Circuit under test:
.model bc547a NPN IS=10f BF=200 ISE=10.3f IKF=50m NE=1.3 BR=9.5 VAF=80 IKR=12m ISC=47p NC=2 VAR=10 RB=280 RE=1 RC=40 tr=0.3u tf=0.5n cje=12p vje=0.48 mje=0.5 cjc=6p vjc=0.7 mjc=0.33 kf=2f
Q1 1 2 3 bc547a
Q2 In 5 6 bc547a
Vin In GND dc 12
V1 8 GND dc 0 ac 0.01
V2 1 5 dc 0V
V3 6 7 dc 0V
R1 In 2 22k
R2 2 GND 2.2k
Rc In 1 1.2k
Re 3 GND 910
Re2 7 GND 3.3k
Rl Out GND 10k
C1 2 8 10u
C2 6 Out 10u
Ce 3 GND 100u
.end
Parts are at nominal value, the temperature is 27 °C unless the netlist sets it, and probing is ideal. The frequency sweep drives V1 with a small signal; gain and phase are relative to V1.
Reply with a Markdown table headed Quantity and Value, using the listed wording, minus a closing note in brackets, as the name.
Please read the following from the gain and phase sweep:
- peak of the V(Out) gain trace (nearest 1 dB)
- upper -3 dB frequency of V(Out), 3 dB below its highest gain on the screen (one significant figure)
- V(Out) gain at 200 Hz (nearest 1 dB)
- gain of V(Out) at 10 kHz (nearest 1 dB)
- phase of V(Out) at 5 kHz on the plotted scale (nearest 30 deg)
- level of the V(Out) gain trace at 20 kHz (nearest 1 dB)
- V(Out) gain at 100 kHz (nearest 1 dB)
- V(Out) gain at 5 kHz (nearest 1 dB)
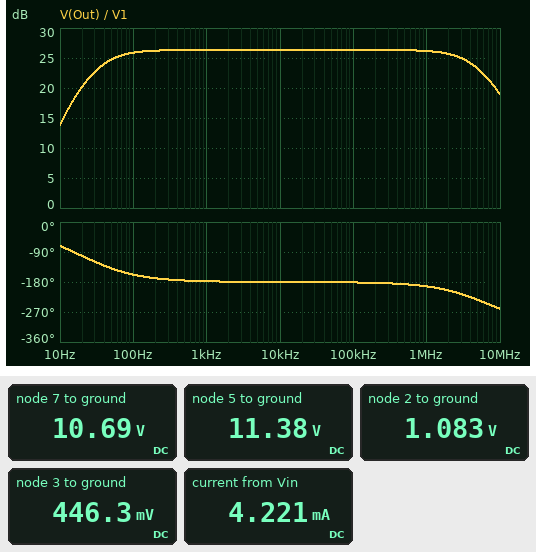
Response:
| Quantity | Value |
|---|---|
| peak of the V(Out) gain trace | 26 dB |
| upper -3 dB frequency of V(Out), 3 dB below its highest gain on the screen | 5 MHz |
| V(Out) gain at 200 Hz | 26 dB |
| gain of V(Out) at 10 kHz | 26 dB |
| phase of V(Out) at 5 kHz on the plotted scale | -180 deg |
| level of the V(Out) gain trace at 20 kHz | 26 dB |
| V(Out) gain at 100 kHz | 26 dB |
| V(Out) gain at 5 kHz | 26 dB |
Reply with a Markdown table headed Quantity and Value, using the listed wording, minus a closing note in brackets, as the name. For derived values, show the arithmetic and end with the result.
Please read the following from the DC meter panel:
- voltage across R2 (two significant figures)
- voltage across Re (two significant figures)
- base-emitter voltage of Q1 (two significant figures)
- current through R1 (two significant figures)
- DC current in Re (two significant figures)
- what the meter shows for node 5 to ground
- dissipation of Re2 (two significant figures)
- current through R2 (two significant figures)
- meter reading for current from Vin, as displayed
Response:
| Quantity | Value |
|---|---|
| voltage across R2 | 1.083 V = 1.1 V |
| voltage across Re | 446.3 mV = 450 mV |
| base-emitter voltage of Q1 | 1.083 V - 446.3 mV = 640 mV |
| current through R1 | (12 V - 1.083 V) / 22 kΩ = 500 µA |
| DC current in Re | (446.3 mV) / 910 Ω = 490 µA |
| what the meter shows for node 5 to ground | 11.38 V |
| dissipation of Re2 | (10.69 V)^2 / 3.3 kΩ = 35 mW |
| current through R2 | (1.083 V) / 2.2 kΩ = 490 µA |
| meter reading for current from Vin, as displayed | 4.221 mA |
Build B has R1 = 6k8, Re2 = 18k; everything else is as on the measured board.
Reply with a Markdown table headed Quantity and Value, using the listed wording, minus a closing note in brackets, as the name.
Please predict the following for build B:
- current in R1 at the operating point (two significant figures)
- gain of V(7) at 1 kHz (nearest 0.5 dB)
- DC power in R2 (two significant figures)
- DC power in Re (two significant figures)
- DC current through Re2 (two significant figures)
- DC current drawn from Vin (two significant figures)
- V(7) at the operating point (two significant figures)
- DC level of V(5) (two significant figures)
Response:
| Quantity | Value |
|---|---|
| current in R1 at the operating point | 1.3 mA |
| gain of V(7) at 1 kHz | 38.0 dB |
| DC power in R2 | 3.8 mW |
| DC power in Re | 5.4 mW |
| DC current through Re2 | 470 µA |
| DC current drawn from Vin | 4.2 mA |
| V(7) at the operating point | 8.5 V |
| DC level of V(5) | 9.1 V |
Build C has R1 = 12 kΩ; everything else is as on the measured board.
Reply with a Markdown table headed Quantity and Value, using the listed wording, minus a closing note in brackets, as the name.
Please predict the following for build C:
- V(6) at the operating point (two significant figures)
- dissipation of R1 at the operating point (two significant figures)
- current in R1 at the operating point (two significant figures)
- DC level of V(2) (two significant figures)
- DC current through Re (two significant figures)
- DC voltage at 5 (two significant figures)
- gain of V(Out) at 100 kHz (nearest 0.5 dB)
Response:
| Quantity | Value |
|---|---|
| V(6) at the operating point | 9.7 V |
| dissipation of R1 at the operating point | 8.6 mW |
| current in R1 at the operating point | 850 µA |
| DC level of V(2) | 1.8 V |
| DC current through Re | 1.3 mA |
| DC voltage at 5 | 10 V |
| gain of V(Out) at 100 kHz | 34.0 dB |
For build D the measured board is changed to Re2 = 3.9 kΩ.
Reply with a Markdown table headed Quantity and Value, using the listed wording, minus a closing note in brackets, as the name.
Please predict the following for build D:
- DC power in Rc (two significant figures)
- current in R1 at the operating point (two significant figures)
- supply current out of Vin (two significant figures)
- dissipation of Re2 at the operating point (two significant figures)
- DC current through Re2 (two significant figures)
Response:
| Quantity | Value |
|---|---|
| DC power in Rc | 310 µW |
| current in R1 at the operating point | 500 µA |
| supply current out of Vin | 3.7 mA |
| dissipation of Re2 at the operating point | 29 mW |
| DC current through Re2 | 2.7 mA |
